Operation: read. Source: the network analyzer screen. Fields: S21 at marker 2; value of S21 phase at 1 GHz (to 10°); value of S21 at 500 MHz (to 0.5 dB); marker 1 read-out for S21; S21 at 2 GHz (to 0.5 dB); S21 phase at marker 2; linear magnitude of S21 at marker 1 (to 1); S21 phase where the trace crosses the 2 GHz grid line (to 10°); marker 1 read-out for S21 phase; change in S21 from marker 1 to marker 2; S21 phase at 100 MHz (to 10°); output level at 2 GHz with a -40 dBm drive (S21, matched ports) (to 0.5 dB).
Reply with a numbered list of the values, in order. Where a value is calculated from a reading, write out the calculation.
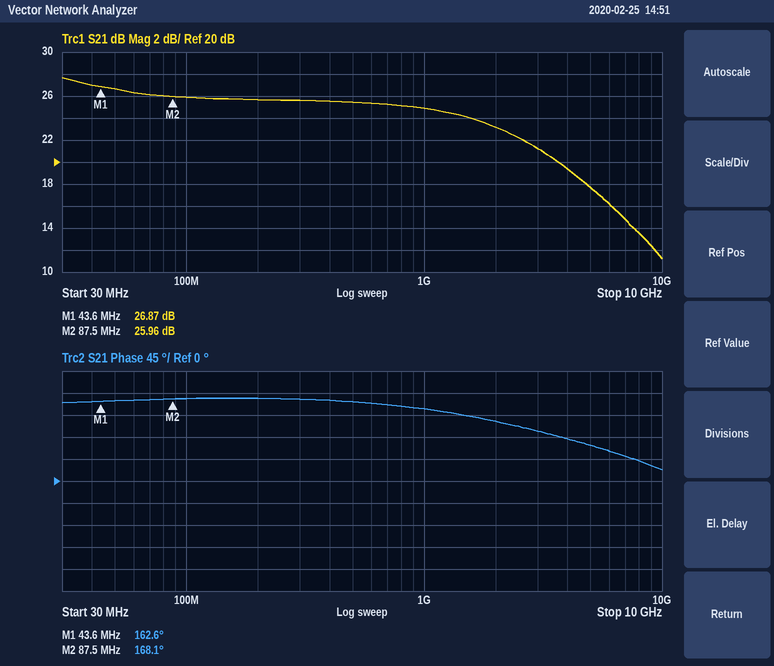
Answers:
1. 25.96 dB
2. 150°
3. 25.5 dB
4. 26.87 dB
5. 23.0 dB
6. 168.1°
7. 10^(26.87/20) ≈ 22
8. 120°
9. 162.6°
10. 25.96 − (26.87) = -0.91 dB
11. 170°
12. -40 dBm + (23.0 dB) = -17.0 dBm
